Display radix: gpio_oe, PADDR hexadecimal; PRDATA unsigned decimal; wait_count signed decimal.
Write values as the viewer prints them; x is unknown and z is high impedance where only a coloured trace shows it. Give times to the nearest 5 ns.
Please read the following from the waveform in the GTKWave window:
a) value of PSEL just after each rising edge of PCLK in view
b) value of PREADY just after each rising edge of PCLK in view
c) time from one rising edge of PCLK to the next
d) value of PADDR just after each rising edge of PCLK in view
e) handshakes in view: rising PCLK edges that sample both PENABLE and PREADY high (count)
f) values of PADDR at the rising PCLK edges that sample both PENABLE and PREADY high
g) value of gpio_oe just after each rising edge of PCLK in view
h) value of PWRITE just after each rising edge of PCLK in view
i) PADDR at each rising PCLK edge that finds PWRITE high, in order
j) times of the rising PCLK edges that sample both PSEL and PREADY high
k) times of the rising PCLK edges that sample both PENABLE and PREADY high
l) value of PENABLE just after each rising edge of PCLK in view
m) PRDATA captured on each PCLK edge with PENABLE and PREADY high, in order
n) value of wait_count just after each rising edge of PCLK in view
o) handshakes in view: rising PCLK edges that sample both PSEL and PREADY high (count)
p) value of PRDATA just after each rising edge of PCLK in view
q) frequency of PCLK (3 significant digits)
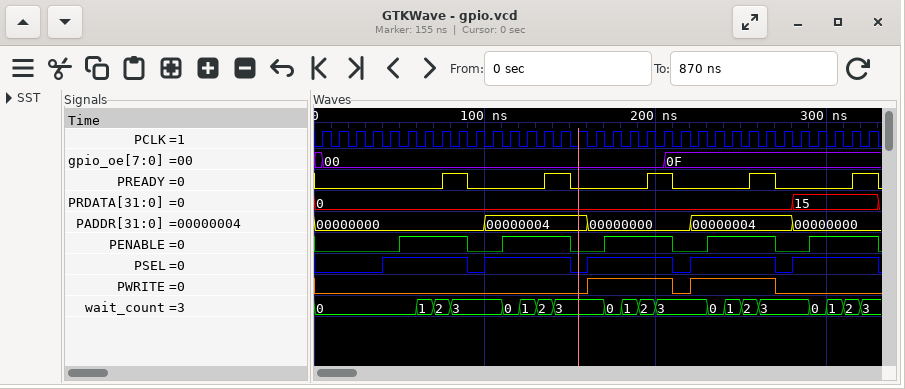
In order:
0 0 0 0 1 1 1 1 1 0 1 1 1 1 1 0 1 1 1 1 1 0 1 1 1 1 1 0 1 1 1 1 1
0 0 0 0 0 0 0 1 1 0 0 0 0 1 1 0 0 0 0 1 1 0 0 0 0 1 1 0 0 0 0 1 1
10 ns
00000000, 00000000, 00000000, 00000000, 00000000, 00000000, 00000000, 00000000, 00000000, 00000000, 00000004, 00000004, 00000004, 00000004, 00000004, 00000004, 00000000, 00000000, 00000000, 00000000, 00000000, 00000000, 00000004, 00000004, 00000004, 00000004, 00000004, 00000004, 00000000, 00000000, 00000000, 00000000, 00000000
5
00000000, 00000004, 00000000, 00000004, 00000000
00, 00, 00, 00, 00, 00, 00, 00, 00, 00, 00, 00, 00, 00, 00, 00, 00, 00, 00, 00, 0F, 0F, 0F, 0F, 0F, 0F, 0F, 0F, 0F, 0F, 0F, 0F, 0F
0 0 0 0 0 0 0 0 0 0 0 0 0 0 0 0 1 1 1 1 1 0 1 1 1 1 1 0 0 0 0 0 0
00000000, 00000000, 00000000, 00000000, 00000000, 00000004, 00000004, 00000004, 00000004, 00000004
85 ns, 145 ns, 205 ns, 265 ns, 325 ns
85 ns, 145 ns, 205 ns, 265 ns, 325 ns
0 0 0 0 0 1 1 1 1 0 0 1 1 1 1 0 0 1 1 1 1 0 0 1 1 1 1 0 0 1 1 1 1
0, 0, 0, 0, 15
0, 0, 0, 0, 0, 0, 1, 2, 3, 3, 3, 0, 1, 2, 3, 3, 3, 0, 1, 2, 3, 3, 3, 0, 1, 2, 3, 3, 3, 0, 1, 2, 3
5
0, 0, 0, 0, 0, 0, 0, 0, 0, 0, 0, 0, 0, 0, 0, 0, 0, 0, 0, 0, 0, 0, 0, 0, 0, 0, 0, 0, 15, 15, 15, 15, 15
100 MHz
